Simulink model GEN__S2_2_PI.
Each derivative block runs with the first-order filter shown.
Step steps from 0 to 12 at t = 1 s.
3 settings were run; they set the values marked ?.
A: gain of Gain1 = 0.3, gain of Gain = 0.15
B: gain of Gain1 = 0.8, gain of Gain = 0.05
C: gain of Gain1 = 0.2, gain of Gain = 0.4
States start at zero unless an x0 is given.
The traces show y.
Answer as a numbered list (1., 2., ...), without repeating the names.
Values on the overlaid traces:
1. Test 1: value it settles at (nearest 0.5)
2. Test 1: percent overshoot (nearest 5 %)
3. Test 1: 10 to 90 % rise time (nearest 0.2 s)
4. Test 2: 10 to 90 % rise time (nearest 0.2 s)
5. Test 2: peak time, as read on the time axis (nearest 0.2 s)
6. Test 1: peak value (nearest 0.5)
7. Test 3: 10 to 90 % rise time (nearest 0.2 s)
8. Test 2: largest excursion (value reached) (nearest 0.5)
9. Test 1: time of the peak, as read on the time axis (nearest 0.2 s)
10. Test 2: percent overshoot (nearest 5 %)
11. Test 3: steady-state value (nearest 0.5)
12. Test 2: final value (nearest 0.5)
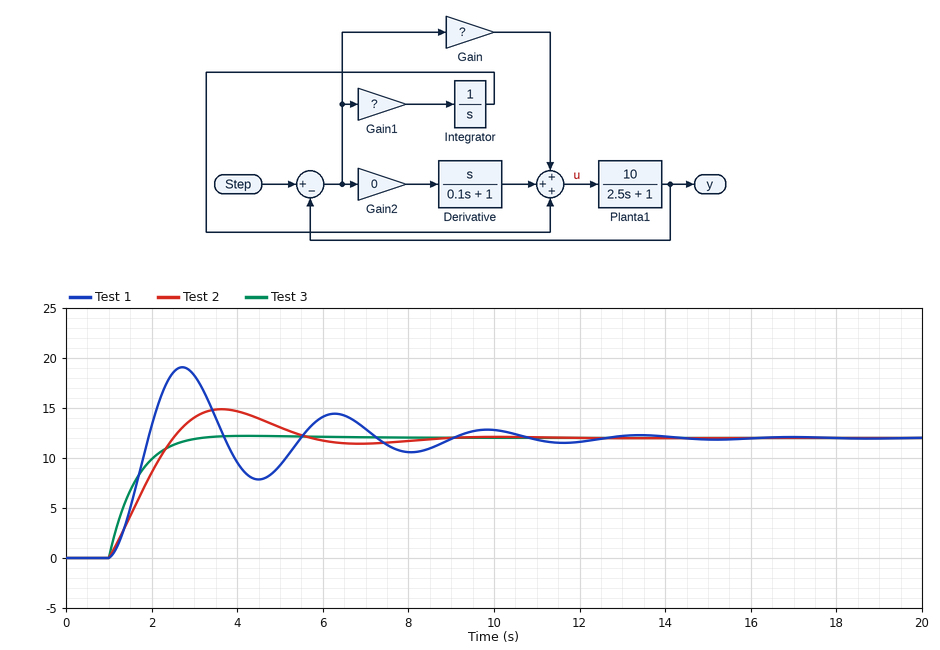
1. 12.0
2. 60 %
3. 0.6 s
4. 1.2 s
5. 3.6 s
6. 19.0
7. 1.2 s
8. 15.0
9. 2.8 s
10. 25 %
11. 12.0
12. 12.0
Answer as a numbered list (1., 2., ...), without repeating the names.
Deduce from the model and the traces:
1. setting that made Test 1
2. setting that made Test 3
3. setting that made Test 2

1. B
2. C
3. A
